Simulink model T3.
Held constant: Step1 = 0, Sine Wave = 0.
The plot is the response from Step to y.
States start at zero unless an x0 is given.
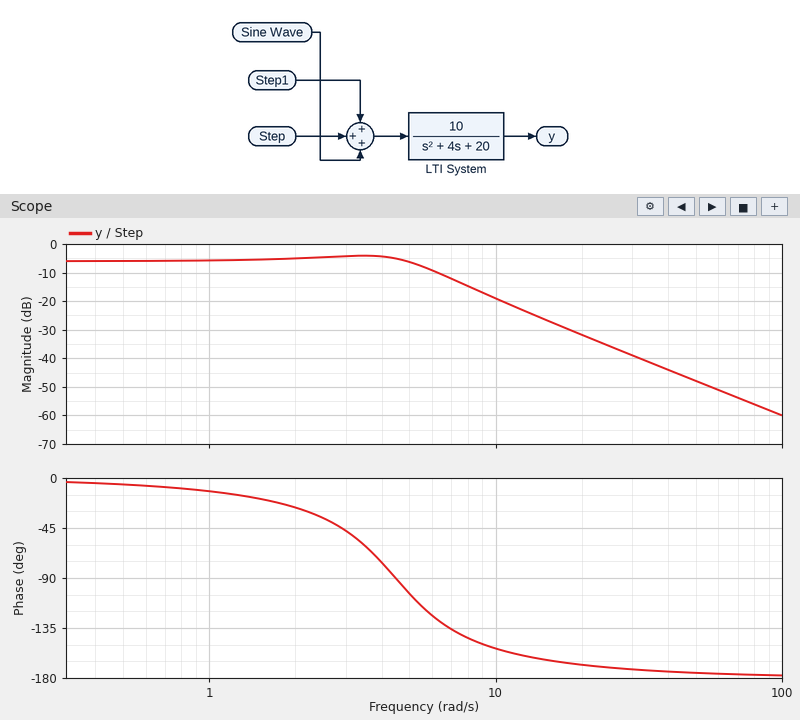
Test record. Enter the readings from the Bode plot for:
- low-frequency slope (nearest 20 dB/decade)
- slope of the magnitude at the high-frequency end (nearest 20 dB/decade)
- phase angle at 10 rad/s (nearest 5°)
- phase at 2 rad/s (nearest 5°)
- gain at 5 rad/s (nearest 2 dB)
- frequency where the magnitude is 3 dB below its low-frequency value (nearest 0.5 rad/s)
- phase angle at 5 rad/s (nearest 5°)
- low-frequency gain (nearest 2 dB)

0 dB/decade
-40 dB/decade
-155°
-25°
-6 dB
6.0 rad/s
-105°
-6 dB
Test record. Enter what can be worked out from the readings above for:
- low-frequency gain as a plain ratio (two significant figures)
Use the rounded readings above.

0.50
